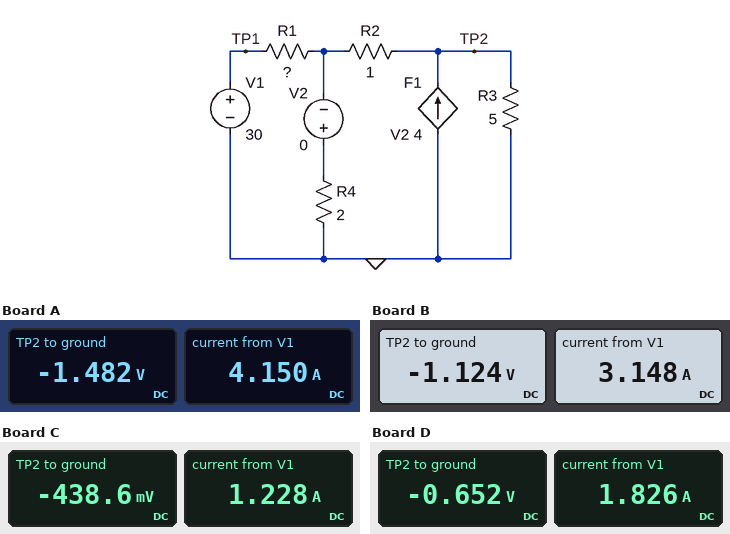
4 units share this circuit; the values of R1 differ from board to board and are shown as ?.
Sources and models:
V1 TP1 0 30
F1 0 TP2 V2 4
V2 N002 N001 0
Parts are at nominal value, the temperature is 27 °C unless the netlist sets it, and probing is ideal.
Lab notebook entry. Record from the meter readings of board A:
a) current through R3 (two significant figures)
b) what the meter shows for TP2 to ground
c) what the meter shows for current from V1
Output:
300 mA
-1.482 V
4.150 A
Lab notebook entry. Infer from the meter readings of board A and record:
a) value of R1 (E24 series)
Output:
6.8 Ω
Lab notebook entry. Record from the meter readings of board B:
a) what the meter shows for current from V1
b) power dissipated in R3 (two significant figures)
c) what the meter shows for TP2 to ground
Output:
3.148 A
250 mW
-1.124 V
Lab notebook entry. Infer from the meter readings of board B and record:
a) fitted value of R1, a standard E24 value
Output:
9.1 Ω
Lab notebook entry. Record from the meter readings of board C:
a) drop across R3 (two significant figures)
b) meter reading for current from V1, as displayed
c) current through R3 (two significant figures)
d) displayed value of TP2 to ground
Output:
440 mV
1.228 A
88 mA
-438.6 mV
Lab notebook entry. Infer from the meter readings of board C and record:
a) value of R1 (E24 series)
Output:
24 Ω
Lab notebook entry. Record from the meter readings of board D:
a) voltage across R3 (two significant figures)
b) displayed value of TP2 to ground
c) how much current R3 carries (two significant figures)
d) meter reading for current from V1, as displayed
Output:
650 mV
-0.652 V
130 mA
1.826 A
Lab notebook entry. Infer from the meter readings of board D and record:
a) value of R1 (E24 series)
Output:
16 Ω
